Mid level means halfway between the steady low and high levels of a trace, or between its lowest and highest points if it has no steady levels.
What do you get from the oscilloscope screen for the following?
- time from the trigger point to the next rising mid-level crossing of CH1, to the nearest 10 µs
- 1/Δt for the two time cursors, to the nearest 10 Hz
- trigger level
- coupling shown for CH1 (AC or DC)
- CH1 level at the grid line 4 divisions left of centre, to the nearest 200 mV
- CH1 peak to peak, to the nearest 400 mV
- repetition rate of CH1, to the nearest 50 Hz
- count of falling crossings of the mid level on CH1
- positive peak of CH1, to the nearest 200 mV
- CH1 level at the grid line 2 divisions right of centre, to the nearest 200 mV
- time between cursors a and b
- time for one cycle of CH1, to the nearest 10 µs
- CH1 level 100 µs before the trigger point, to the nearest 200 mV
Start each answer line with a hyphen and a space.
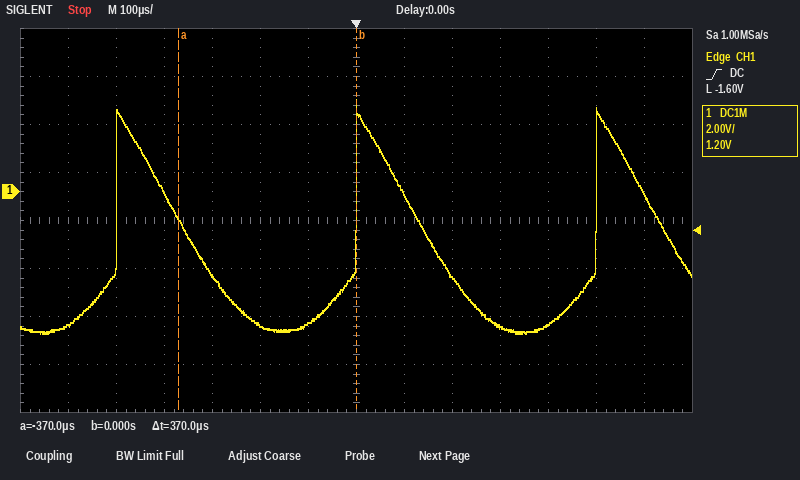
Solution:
- 500 µs
- 2.70 kHz
- -1.60 V
- DC
- 0.0 V
- 9.6 V
- 2.00 kHz
- 3
- 3.8 V
- -3.6 V
- 370 µs
- 500 µs
- -5.4 V
